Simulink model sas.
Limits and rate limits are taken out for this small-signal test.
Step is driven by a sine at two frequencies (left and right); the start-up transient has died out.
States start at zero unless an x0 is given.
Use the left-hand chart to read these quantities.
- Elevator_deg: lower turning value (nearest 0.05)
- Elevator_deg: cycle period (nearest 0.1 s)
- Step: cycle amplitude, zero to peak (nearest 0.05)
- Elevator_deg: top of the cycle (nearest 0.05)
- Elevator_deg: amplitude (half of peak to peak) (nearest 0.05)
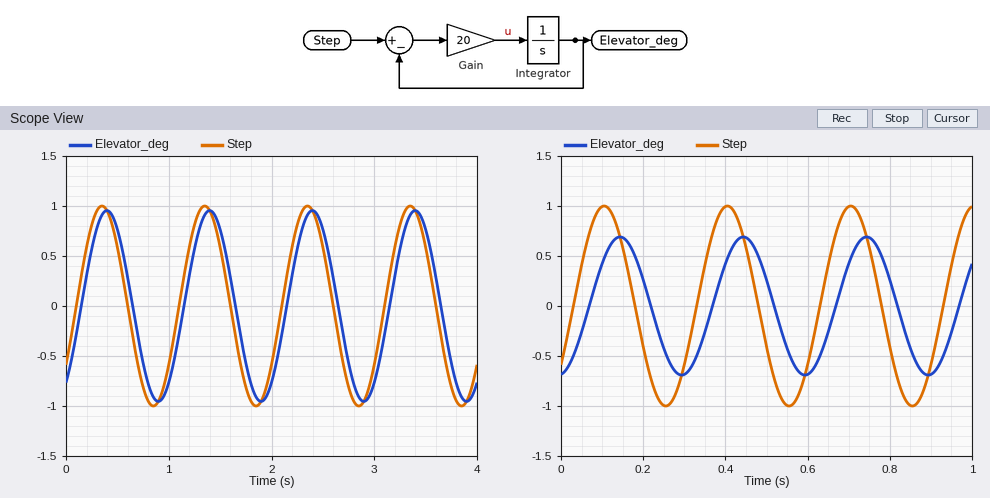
-0.95
1.0 s
1.00
0.95
0.95
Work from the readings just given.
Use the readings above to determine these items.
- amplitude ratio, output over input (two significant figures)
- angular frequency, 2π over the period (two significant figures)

0.95
6.3 rad/s
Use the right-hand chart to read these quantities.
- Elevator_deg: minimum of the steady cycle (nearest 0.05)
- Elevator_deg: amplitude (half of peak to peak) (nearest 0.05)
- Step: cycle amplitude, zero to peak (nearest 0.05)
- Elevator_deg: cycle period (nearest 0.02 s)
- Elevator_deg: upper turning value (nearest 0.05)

-0.70
0.70
1.00
0.30 s
0.70
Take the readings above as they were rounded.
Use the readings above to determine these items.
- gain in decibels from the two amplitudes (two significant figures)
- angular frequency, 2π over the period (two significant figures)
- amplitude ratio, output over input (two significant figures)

-3.1 dB
21 rad/s
0.70
